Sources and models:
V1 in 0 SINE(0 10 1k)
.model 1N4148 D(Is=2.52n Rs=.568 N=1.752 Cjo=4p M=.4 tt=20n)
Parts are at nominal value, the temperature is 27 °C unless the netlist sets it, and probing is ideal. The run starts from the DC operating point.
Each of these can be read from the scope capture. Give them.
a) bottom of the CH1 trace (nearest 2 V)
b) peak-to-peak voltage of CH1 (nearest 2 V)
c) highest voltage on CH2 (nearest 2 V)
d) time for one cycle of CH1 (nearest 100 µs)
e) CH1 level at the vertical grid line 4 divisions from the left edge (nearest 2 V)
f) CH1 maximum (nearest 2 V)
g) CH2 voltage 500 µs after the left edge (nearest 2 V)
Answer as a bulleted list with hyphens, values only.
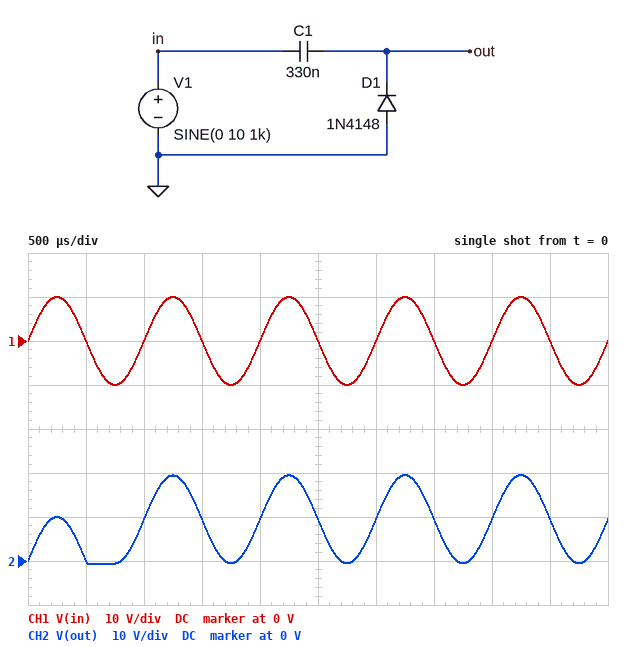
- -10 V
- 20 V
- 20 V
- 1.0 ms
- 0 V
- 10 V
- 0 V
